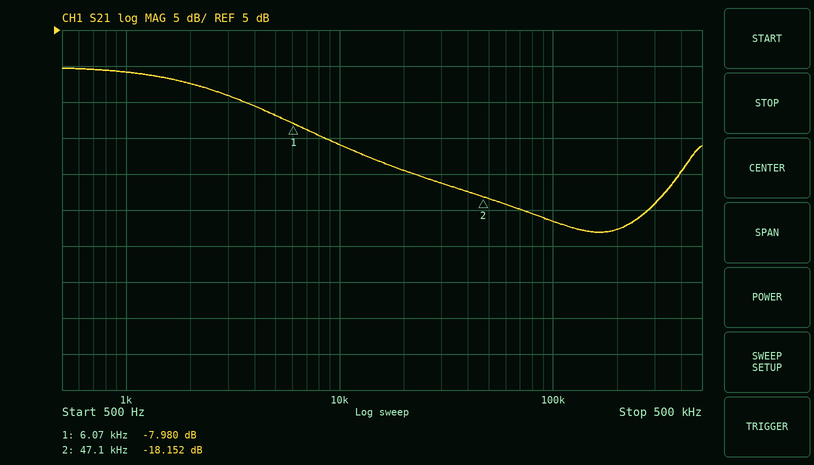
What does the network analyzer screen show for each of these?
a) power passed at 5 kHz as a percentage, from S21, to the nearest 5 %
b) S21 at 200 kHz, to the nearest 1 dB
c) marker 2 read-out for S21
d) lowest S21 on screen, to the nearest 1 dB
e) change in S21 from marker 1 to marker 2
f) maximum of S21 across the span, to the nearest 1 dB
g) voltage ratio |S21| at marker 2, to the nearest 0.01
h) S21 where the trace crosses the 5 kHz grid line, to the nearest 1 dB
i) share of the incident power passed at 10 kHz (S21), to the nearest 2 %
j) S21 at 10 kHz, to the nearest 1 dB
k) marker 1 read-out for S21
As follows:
20 %
-23 dB
-18.152 dB
-23 dB
-10.172 dB
0 dB
0.12
-7 dB
8 %
-11 dB
-7.980 dB
